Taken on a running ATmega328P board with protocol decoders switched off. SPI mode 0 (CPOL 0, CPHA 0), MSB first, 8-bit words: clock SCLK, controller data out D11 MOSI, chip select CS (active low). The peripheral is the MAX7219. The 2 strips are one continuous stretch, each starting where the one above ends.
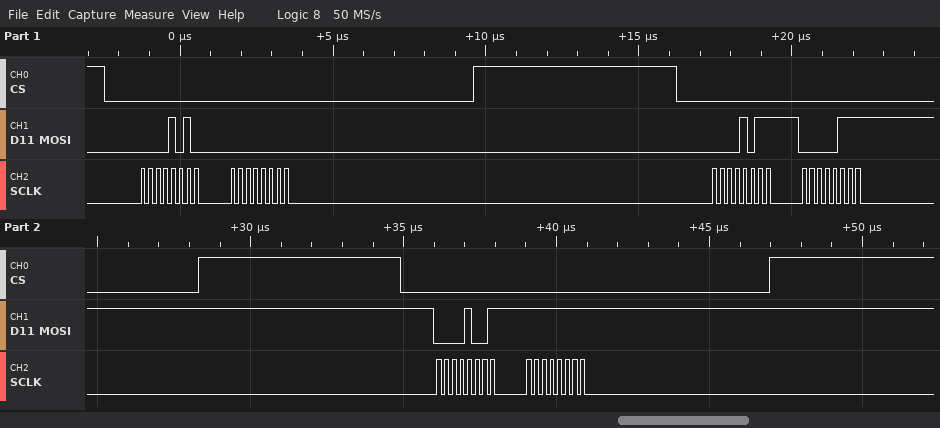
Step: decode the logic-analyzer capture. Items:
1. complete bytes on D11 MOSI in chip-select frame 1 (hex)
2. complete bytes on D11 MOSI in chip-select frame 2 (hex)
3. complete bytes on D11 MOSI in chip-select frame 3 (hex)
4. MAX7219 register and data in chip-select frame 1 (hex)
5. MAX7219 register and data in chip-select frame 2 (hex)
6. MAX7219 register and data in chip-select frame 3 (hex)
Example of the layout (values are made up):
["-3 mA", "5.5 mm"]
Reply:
["0A 00", "0B 07", "09 FF", "register 0xA, data 0x00", "register 0xB, data 0x07", "register 0x9, data 0xFF"]
